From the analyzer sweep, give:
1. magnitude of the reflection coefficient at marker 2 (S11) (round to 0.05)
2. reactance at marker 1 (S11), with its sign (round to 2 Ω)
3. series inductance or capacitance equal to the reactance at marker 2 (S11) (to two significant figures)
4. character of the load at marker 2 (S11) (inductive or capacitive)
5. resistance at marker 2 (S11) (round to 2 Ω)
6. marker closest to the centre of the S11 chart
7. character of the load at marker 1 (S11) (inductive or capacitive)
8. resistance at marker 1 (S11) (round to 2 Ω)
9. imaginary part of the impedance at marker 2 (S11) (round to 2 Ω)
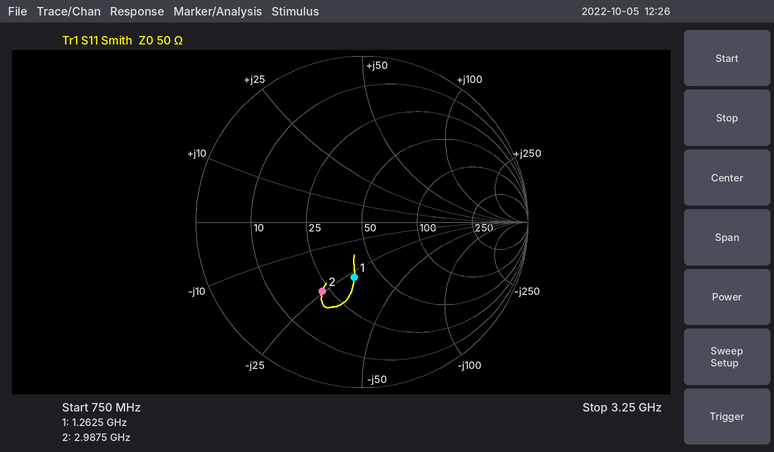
0.50
-28 Ω
2.2 pF
capacitive
22 Ω
marker 1
capacitive
36 Ω
-24 Ω
